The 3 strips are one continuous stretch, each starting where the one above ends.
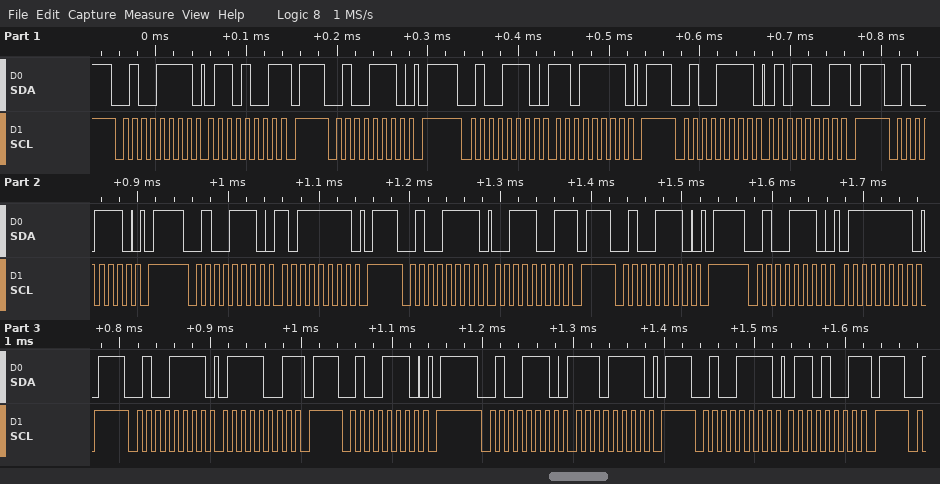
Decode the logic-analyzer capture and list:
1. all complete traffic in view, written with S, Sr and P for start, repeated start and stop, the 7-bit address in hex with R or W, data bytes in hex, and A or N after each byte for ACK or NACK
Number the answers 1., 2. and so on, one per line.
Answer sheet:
1. S 27R A 69 N P S 27W A P S 27W A DF A P S 27R A 59 N P S 27W A P S 27W A BF A P S 27R A 39 N P S 27W A P S 27W A 7F A P S 27R A 79 N P S 27W A P S 27W A EF A P S 27R A 69 N P
